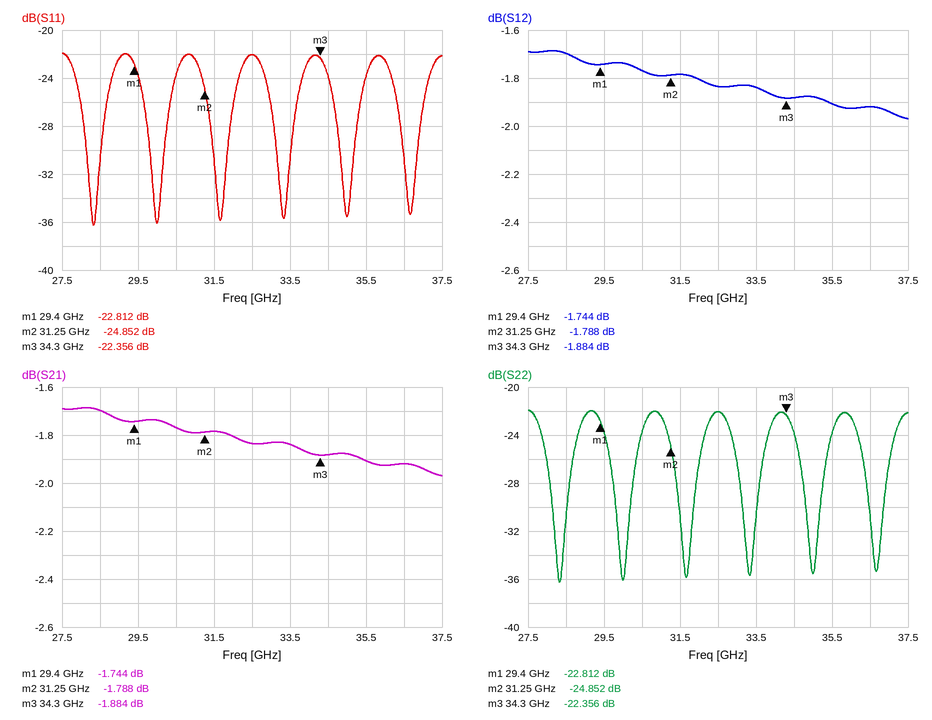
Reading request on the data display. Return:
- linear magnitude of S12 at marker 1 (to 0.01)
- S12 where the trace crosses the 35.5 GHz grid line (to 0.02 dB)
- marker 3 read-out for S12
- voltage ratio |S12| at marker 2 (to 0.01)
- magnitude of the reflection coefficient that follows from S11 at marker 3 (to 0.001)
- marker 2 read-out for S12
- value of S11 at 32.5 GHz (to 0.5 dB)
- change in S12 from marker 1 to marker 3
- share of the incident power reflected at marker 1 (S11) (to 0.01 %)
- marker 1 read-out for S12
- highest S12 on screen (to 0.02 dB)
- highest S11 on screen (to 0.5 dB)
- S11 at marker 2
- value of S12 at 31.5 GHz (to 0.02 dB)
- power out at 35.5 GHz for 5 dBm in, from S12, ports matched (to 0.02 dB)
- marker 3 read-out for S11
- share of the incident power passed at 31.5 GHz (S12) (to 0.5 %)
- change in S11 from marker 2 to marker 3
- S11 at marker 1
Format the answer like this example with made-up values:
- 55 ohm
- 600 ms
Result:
- 0.82
- -1.90 dB
- -1.884 dB
- 0.81
- 0.076
- -1.788 dB
- -22.0 dB
- -0.140 dB
- 0.52 %
- -1.744 dB
- -1.68 dB
- -22.0 dB
- -24.852 dB
- -1.78 dB
- 3.10 dBm
- -22.356 dB
- 66.5 %
- 2.496 dB
- -22.812 dB
